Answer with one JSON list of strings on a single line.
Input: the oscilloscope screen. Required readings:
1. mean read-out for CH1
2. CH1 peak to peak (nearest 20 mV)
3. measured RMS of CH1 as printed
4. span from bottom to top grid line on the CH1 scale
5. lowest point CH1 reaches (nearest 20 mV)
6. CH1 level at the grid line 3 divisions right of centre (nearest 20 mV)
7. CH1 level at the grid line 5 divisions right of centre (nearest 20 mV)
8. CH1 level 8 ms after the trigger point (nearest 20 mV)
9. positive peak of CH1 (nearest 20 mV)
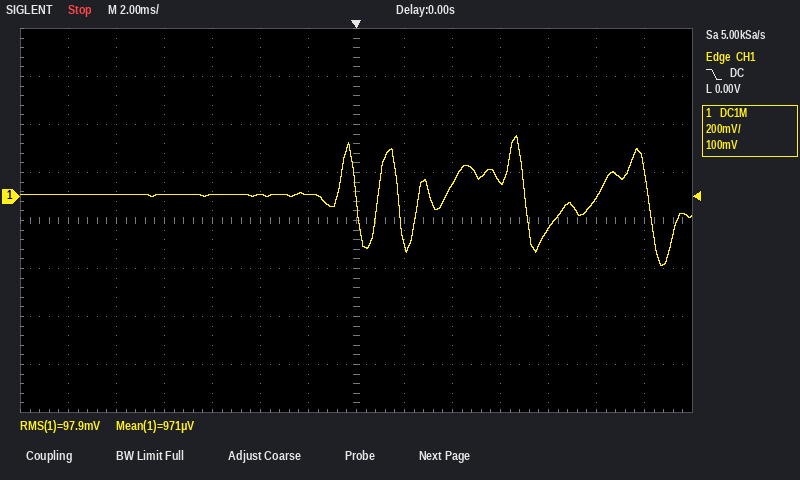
["971 µV", "540 mV", "97.9 mV", "1.6 V", "-280 mV", "60 mV", "0 mV", "-140 mV", "260 mV"]
